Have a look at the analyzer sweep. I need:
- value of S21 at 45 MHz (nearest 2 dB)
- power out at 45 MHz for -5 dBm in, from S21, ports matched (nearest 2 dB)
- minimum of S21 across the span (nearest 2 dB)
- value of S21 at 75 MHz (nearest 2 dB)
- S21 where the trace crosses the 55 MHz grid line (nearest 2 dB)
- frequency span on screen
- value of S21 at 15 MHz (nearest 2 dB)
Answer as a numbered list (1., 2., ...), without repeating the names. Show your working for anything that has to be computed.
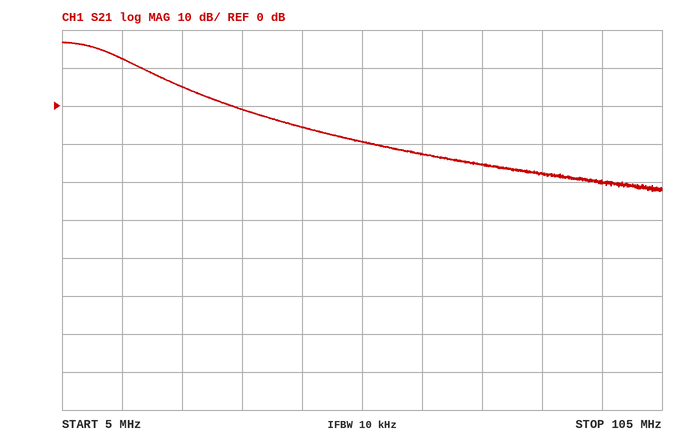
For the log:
1. -6 dB
2. -5 dBm + (-6 dB) = -10 dBm
3. -22 dB
4. -16 dB
5. -10 dB
6. 100 MHz
7. 12 dB
